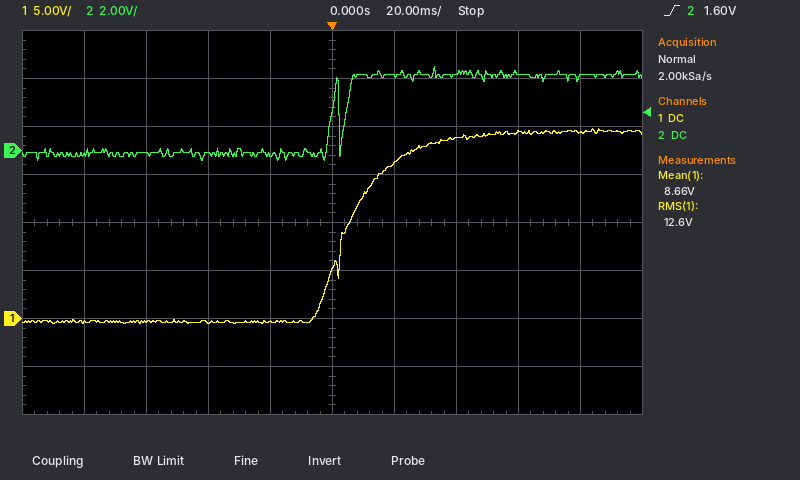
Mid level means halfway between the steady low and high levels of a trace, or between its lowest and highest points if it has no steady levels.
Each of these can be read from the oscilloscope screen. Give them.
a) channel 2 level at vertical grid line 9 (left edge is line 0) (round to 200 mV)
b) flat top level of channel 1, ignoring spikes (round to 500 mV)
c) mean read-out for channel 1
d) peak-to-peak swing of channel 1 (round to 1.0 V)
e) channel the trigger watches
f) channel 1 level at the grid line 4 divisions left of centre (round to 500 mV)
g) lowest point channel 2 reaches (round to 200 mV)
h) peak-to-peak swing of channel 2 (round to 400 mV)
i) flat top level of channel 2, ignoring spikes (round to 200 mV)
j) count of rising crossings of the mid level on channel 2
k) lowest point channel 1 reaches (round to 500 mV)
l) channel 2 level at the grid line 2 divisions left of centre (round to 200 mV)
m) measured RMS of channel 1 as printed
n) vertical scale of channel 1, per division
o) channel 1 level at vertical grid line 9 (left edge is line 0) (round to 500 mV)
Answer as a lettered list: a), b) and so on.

a) 3.0 V
b) 19.5 V
c) 8.66 V
d) 20.0 V
e) channel 2
f) -500 mV
g) -400 mV
h) 4.0 V
i) 3.2 V
j) 2
k) -500 mV
l) -200 mV
m) 12.6 V
n) 5 V
o) 19.5 V
